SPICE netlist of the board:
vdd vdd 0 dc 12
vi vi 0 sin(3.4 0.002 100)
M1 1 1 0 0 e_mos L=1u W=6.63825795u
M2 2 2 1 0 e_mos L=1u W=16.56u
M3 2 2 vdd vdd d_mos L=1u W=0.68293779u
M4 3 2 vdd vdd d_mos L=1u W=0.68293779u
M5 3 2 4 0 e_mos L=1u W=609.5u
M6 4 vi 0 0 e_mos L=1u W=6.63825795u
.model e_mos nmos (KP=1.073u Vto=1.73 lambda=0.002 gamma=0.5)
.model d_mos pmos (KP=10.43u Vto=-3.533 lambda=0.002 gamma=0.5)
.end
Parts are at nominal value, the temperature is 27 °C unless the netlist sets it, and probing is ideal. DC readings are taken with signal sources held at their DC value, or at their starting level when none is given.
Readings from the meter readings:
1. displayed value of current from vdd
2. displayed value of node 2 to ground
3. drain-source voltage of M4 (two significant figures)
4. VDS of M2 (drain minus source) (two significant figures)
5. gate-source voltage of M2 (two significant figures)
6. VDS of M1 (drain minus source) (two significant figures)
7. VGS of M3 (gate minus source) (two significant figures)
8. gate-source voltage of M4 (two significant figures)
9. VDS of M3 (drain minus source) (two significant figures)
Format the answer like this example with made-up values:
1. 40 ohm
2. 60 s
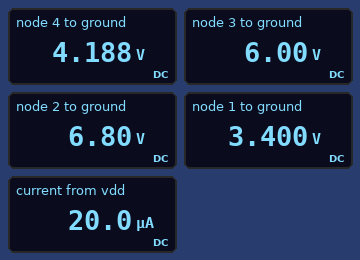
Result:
1. 20.0 µA
2. 6.80 V
3. -6.0 V
4. 3.4 V
5. 3.4 V
6. 3.4 V
7. -5.2 V
8. -5.2 V
9. -5.2 V
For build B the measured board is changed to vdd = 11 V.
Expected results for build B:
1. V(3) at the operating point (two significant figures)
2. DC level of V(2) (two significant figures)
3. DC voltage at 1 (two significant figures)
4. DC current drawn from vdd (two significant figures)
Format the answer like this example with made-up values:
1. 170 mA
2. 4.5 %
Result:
1. 650 mV
2. 6.2 V
3. 3.0 V
4. 12 µA
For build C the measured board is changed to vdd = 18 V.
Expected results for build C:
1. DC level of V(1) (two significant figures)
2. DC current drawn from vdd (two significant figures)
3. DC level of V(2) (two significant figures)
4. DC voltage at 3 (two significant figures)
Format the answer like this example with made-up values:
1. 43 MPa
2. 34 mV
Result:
1. 5.6 V
2. 64 µA
3. 11 V
4. 18 V
